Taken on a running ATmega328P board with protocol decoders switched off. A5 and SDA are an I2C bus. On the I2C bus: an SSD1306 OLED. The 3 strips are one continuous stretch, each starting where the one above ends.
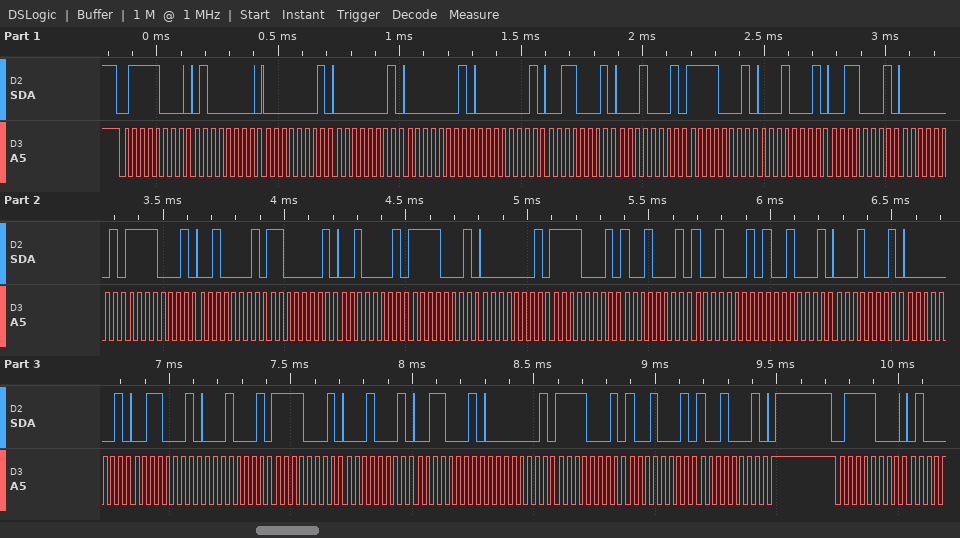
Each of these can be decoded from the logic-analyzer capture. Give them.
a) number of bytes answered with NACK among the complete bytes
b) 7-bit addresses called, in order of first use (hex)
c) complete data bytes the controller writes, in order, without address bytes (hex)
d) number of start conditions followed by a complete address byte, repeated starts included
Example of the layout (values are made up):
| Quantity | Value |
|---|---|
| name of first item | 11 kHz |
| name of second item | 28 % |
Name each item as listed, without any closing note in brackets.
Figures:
| Quantity | Value |
|---|---|
| number of bytes answered with NACK among the complete bytes | 0 |
| 7-bit addresses called, in order of first use | 0x3C |
| complete data bytes the controller writes, in order, without address bytes | 40 01 01 01 01 31 11 F1 11 31 01 F1 21 C1 21 F1 01 F1 91 91 91 11 01 31 11 F1 11 31 01 F1 91 91 |
| number of start conditions followed by a complete address byte, repeated starts included | 2 |
